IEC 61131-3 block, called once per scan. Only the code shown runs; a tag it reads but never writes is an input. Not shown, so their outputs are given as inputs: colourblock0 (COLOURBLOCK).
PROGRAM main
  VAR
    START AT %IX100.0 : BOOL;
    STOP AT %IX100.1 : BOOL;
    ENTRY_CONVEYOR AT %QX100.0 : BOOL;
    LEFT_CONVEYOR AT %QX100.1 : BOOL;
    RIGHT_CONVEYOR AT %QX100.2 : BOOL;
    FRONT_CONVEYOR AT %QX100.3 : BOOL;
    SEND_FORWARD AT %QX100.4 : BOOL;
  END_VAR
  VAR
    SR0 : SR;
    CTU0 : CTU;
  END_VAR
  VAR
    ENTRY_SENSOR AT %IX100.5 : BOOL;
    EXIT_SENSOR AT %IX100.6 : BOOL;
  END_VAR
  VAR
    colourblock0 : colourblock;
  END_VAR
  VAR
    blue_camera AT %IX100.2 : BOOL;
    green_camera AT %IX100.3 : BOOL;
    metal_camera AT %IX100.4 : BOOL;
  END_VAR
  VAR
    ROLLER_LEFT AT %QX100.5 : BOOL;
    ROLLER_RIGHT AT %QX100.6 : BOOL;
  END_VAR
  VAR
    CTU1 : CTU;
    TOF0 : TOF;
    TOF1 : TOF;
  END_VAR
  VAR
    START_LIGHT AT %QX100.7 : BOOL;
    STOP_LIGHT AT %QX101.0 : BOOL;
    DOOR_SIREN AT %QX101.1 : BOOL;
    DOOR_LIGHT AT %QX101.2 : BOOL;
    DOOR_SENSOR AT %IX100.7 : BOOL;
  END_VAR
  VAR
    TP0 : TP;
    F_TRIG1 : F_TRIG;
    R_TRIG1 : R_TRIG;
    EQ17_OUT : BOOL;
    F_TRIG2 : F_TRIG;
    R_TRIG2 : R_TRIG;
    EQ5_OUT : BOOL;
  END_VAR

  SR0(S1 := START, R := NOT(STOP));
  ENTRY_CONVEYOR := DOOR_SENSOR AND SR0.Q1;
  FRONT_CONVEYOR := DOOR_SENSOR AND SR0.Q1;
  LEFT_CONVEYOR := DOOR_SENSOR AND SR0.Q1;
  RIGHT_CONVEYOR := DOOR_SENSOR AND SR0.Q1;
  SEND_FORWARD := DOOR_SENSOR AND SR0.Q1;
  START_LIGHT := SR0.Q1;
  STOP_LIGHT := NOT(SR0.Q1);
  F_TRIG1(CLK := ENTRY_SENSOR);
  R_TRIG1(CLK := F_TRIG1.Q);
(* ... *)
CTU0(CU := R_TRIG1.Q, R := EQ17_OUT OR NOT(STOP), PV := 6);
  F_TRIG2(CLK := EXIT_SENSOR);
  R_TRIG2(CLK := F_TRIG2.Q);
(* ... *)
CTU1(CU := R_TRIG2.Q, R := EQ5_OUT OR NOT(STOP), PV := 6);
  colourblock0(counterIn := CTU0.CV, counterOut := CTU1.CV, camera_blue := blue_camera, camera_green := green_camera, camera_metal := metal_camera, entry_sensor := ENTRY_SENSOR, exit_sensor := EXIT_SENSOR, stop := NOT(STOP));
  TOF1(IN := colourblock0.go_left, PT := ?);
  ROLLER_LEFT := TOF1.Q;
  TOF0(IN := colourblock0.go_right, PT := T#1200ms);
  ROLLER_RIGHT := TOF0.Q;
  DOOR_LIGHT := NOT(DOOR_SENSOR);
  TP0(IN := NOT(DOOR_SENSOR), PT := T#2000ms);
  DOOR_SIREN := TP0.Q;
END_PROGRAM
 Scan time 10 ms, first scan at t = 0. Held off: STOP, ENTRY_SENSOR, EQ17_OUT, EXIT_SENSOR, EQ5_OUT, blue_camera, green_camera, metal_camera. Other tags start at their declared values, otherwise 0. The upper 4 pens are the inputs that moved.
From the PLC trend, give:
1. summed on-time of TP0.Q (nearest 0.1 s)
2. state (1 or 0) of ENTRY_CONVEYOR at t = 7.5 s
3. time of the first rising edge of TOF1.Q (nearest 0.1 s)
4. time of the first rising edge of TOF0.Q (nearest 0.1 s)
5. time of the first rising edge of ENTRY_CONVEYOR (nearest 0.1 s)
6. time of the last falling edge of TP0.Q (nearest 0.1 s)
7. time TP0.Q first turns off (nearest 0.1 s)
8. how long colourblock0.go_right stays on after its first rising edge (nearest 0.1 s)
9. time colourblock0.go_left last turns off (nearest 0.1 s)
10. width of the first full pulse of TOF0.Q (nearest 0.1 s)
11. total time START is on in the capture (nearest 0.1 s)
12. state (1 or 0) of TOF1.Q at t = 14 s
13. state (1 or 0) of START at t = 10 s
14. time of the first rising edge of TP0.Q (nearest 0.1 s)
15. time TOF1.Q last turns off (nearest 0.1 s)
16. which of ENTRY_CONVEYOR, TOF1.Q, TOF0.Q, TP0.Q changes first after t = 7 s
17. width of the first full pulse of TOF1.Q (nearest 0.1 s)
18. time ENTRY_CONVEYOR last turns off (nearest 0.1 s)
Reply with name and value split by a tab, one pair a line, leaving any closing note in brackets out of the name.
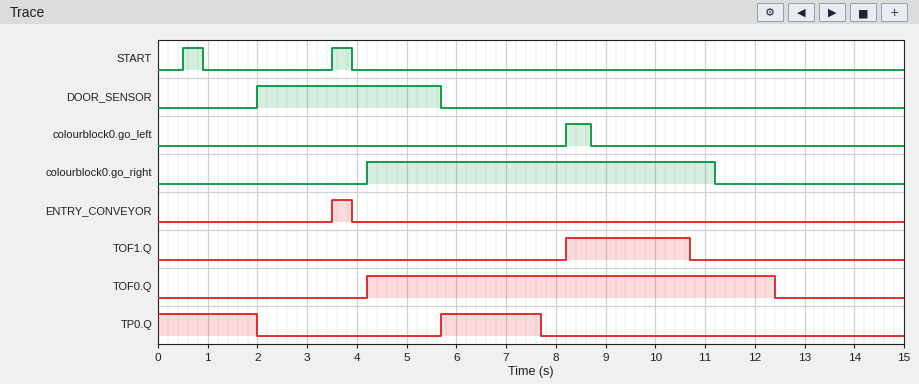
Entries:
summed on-time of TP0.Q	4.0 s
state (1 or 0) of ENTRY_CONVEYOR at t = 7.5 s	0
time of the first rising edge of TOF1.Q	8.2 s
time of the first rising edge of TOF0.Q	4.2 s
time of the first rising edge of ENTRY_CONVEYOR	3.5 s
time of the last falling edge of TP0.Q	7.7 s
time TP0.Q first turns off	2.0 s
how long colourblock0.go_right stays on after its first rising edge	7.0 s
time colourblock0.go_left last turns off	8.7 s
width of the first full pulse of TOF0.Q	8.2 s
total time START is on in the capture	0.8 s
state (1 or 0) of TOF1.Q at t = 14 s	0
state (1 or 0) of START at t = 10 s	0
time of the first rising edge of TP0.Q	5.7 s
time TOF1.Q last turns off	10.7 s
which of ENTRY_CONVEYOR, TOF1.Q, TOF0.Q, TP0.Q changes first after t = 7 s	TP0.Q
width of the first full pulse of TOF1.Q	2.5 s
time ENTRY_CONVEYOR last turns off	3.9 s
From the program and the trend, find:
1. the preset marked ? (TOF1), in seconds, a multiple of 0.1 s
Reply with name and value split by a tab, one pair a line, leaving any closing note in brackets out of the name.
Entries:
the preset marked ? (TOF1), in seconds, a multiple of 0.1 s	2.0 s
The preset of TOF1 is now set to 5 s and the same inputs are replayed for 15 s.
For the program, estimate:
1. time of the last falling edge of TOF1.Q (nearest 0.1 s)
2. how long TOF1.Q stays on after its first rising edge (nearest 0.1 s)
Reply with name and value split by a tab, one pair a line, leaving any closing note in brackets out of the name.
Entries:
time of the last falling edge of TOF1.Q	13.7 s
how long TOF1.Q stays on after its first rising edge	5.5 s
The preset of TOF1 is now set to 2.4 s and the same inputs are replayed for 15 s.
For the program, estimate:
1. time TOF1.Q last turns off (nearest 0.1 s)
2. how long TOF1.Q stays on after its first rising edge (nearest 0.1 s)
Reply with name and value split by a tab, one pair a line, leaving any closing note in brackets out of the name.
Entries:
time TOF1.Q last turns off	11.1 s
how long TOF1.Q stays on after its first rising edge	2.9 s
